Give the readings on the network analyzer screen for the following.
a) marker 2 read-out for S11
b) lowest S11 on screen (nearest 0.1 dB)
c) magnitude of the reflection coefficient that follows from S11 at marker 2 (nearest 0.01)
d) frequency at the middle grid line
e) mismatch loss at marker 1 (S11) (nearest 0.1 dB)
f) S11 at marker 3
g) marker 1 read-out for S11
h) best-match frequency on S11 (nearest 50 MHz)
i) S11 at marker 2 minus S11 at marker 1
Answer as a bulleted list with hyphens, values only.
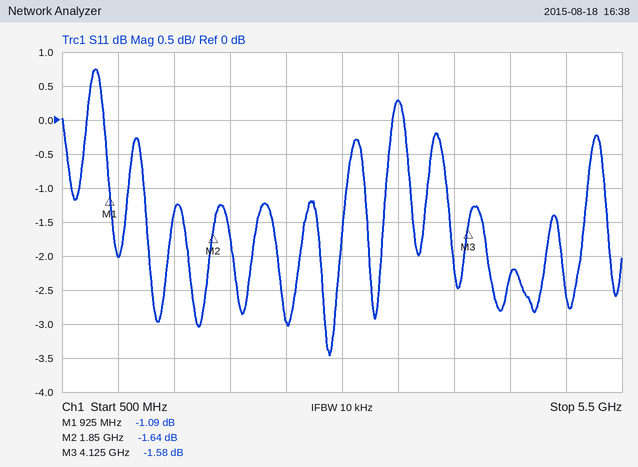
- -1.64 dB
- -3.5 dB
- 0.83
- 3 GHz
- 6.5 dB
- -1.58 dB
- -1.09 dB
- 2.90 GHz
- -0.55 dB
